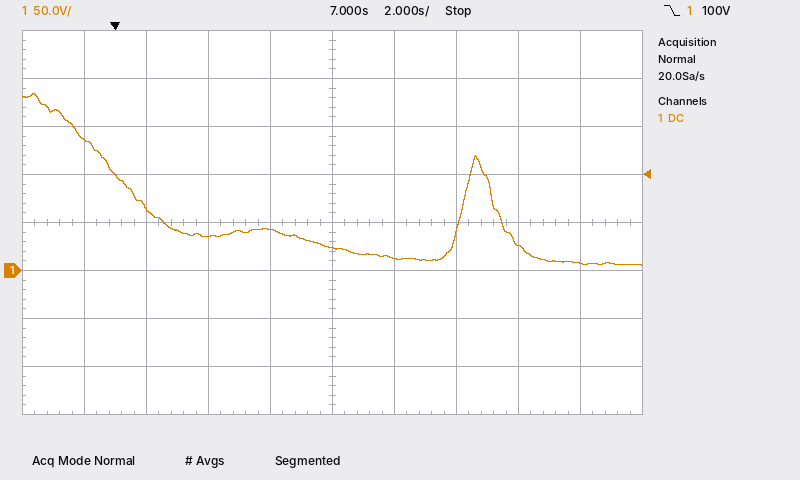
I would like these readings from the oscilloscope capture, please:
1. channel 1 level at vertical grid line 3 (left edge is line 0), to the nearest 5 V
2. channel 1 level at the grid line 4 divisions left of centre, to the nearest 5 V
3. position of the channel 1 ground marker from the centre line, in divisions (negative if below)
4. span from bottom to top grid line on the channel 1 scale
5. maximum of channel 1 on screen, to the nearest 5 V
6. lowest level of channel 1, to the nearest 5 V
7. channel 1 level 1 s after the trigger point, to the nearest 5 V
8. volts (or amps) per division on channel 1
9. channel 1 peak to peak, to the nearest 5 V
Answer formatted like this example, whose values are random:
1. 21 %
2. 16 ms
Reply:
1. 35 V
2. 135 V
3. -1.0 div
4. 400 V
5. 185 V
6. 5 V
7. 65 V
8. 50 V
9. 180 V
